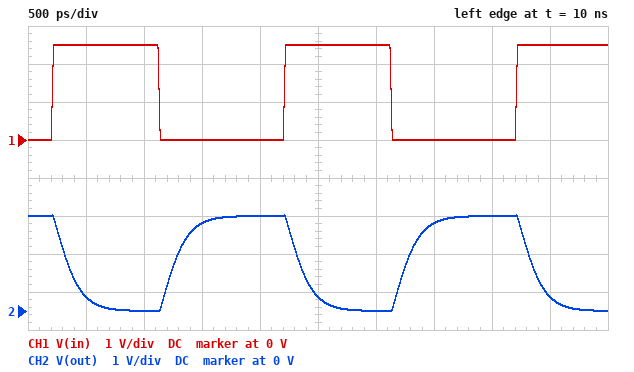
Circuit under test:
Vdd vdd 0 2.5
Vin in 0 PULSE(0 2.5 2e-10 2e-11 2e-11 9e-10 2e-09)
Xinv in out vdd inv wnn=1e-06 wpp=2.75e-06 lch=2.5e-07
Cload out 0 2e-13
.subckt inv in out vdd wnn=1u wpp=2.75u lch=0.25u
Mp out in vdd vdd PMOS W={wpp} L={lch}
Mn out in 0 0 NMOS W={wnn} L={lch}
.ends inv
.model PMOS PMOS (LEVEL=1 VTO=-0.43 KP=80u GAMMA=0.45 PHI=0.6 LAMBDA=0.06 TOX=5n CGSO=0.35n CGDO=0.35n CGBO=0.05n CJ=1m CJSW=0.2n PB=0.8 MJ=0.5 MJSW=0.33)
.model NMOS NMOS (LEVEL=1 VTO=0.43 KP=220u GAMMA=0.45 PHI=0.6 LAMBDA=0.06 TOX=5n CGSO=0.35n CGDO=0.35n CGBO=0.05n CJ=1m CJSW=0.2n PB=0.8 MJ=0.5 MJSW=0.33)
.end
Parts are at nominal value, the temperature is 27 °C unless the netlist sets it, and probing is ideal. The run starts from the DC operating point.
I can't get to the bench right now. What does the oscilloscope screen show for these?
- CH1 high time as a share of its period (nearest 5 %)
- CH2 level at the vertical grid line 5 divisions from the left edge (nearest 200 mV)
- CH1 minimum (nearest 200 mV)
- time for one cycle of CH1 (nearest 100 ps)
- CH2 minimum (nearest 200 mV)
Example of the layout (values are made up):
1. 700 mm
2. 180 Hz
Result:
1. 45 %
2. 400 mV
3. 0 V
4. 2.0 ns
5. 0 V
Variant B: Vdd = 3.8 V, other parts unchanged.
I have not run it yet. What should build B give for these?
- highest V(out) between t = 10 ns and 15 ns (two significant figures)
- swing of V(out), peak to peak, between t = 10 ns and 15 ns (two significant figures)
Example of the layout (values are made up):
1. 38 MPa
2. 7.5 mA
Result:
1. 3.8 V
2. 3.6 V
